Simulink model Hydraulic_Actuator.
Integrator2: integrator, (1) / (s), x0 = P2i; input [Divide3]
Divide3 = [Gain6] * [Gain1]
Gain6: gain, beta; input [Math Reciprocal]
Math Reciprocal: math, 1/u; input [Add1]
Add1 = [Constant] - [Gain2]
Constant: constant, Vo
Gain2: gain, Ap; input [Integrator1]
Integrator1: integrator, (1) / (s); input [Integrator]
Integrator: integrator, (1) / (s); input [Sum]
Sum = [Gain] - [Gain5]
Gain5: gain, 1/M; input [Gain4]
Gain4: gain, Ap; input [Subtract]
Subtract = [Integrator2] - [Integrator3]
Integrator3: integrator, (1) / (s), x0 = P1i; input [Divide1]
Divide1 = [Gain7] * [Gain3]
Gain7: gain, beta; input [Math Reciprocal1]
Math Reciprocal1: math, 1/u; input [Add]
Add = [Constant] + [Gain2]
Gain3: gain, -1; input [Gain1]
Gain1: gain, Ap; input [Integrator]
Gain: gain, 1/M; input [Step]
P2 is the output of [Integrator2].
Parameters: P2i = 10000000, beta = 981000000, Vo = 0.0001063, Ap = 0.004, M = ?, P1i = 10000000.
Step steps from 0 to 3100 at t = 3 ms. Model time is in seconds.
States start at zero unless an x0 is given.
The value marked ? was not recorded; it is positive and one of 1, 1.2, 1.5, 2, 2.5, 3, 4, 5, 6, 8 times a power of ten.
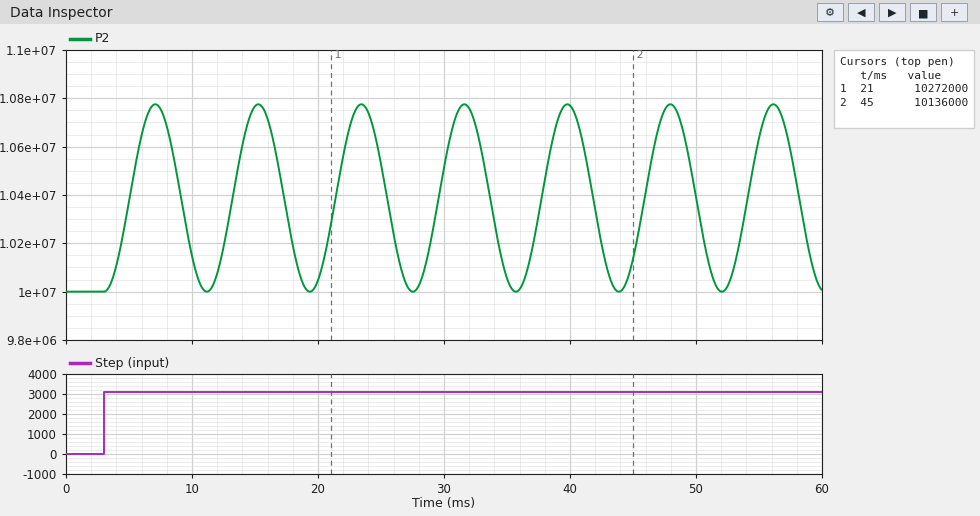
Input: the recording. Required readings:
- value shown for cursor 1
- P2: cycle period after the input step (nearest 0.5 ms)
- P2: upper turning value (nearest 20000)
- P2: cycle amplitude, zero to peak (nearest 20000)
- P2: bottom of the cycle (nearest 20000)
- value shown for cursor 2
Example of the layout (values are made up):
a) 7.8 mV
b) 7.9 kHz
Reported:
a) 10272000
b) 8.0 ms
c) 10780000
d) 380000
e) 10000000
f) 10136000
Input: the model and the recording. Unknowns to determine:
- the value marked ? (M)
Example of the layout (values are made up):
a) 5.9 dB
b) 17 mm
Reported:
a) 500
